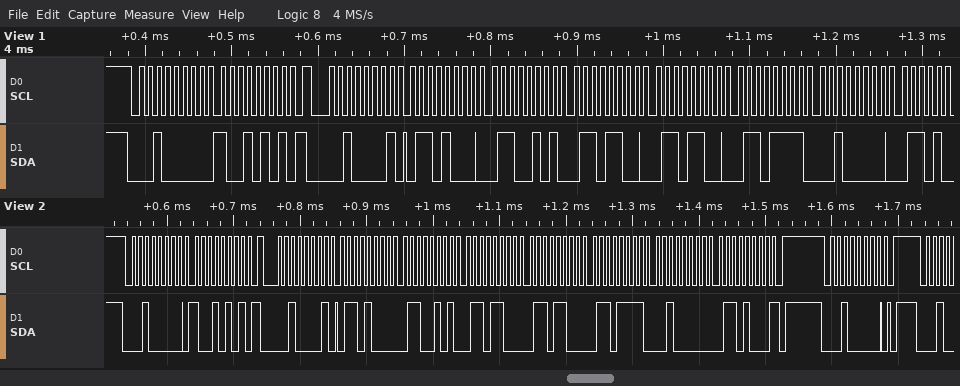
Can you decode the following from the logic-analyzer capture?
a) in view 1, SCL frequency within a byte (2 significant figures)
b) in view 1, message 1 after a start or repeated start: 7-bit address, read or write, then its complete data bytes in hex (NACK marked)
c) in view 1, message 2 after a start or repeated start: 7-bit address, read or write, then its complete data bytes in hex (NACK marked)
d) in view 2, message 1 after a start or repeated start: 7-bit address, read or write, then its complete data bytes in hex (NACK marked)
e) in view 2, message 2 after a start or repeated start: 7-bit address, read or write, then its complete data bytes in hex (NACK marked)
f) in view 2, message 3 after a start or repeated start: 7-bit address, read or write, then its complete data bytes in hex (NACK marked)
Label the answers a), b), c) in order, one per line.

a) 100 kHz
b) 0x10 write: 95
c) 0x10 read: 68 65 6C 6C 6F 20
d) 0x10 write: 95
e) 0x10 read: 68 65 6C 6C 6F 20 68 NACK
f) 0x10 write
